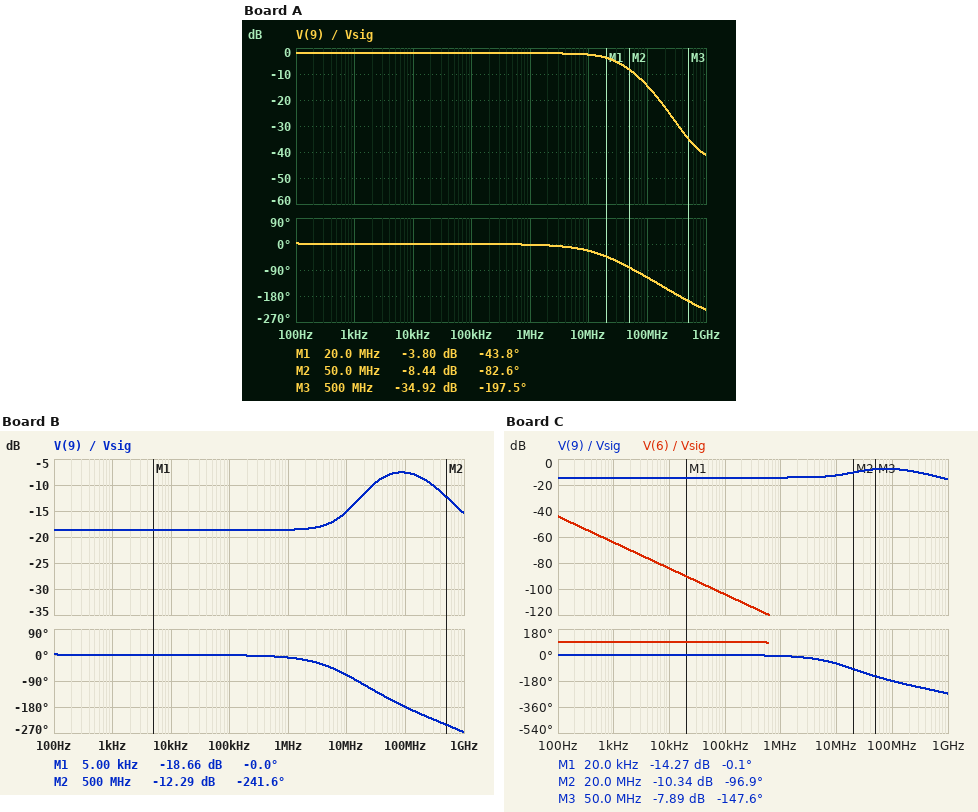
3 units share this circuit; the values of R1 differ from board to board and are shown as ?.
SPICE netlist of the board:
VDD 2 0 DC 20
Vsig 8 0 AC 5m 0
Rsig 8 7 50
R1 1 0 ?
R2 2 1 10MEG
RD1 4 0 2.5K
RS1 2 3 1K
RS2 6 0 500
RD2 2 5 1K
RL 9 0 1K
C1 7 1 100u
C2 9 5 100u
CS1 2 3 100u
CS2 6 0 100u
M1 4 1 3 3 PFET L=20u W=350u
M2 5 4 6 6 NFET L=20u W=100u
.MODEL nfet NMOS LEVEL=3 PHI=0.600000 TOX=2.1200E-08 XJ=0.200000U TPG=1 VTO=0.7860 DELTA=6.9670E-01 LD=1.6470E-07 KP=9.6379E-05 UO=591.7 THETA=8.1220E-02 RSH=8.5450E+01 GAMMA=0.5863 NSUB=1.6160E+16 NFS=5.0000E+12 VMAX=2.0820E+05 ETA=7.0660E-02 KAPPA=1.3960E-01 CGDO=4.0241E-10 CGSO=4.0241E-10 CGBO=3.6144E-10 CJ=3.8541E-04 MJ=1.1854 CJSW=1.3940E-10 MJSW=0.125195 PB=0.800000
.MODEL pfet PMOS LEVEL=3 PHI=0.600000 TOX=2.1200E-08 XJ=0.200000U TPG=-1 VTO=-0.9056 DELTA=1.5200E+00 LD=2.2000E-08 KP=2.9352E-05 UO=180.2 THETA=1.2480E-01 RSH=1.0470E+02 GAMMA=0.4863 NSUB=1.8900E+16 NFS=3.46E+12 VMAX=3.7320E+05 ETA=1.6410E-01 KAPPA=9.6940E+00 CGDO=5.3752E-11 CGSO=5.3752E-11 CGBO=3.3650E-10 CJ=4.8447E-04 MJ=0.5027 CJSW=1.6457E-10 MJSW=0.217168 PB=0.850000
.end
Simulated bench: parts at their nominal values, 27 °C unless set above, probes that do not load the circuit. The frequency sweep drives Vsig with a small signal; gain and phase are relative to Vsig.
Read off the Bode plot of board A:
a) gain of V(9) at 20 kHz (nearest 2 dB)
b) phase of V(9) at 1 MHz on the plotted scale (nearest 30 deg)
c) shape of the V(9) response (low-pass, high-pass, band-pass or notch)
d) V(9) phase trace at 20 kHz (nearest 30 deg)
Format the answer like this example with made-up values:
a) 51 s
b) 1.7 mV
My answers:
a) -2 dB
b) 0 deg
c) low-pass
d) 0 deg
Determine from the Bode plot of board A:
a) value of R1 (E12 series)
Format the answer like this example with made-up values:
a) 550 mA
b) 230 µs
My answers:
a) 22 MΩ
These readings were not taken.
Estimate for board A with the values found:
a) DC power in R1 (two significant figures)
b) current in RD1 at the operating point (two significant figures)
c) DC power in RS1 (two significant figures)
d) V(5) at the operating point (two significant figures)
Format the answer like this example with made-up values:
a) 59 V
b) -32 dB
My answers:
a) 8.6 µW
b) 1.8 mA
c) 3.1 mW
d) 19 V
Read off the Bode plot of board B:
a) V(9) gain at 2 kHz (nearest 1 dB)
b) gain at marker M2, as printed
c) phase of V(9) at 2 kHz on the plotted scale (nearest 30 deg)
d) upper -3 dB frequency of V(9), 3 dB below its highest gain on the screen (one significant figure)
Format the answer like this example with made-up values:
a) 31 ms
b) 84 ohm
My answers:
a) -19 dB
b) -12.29 dB
c) 0 deg
d) 300 MHz
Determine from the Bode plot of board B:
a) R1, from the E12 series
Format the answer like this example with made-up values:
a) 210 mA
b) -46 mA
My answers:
a) 3.3 MΩ
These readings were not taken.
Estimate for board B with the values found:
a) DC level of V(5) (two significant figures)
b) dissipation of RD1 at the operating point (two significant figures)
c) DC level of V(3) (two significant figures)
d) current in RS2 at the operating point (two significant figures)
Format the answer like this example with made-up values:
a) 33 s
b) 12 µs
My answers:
a) 14 V
b) 55 mW
c) 15 V
d) 6.4 mA
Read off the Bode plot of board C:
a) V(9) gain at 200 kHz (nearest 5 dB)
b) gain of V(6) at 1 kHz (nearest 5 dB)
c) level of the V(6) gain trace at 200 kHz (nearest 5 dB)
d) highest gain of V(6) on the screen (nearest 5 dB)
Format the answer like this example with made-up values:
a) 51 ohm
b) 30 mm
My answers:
a) -15 dB
b) -65 dB
c) -110 dB
d) -45 dB
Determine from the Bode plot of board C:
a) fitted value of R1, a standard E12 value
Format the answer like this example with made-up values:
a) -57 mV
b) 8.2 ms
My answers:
a) 4.7 MΩ
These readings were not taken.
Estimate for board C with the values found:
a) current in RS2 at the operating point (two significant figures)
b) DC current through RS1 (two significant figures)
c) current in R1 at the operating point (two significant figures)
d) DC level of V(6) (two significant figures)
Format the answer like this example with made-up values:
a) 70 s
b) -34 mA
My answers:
a) 6.2 mA
b) 4.6 mA
c) 1.4 µA
d) 3.1 V
